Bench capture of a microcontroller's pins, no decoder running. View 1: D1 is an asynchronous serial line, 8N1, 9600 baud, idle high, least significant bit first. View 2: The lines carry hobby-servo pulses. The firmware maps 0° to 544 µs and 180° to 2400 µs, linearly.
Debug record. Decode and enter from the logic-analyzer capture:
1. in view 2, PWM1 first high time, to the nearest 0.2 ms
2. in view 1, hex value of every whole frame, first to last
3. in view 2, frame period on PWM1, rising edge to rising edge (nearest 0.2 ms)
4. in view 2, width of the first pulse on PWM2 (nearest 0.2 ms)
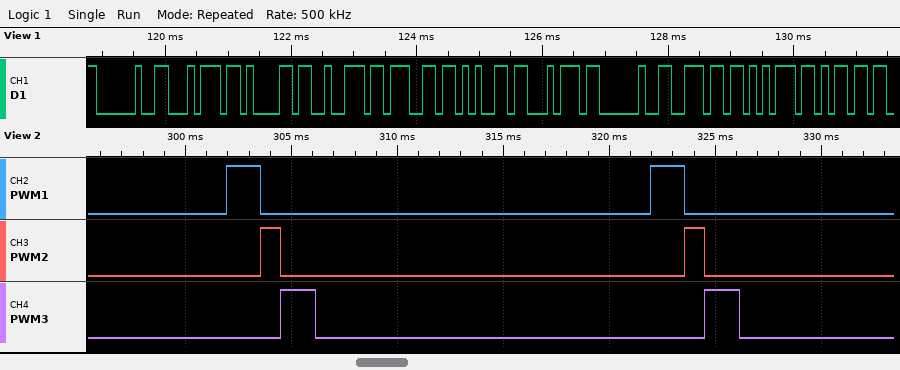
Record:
1.6 ms
0x20 0x74 0x61 0x72 0x67 0x65 0x74 0x20 0x6E 0x75 0x6D
20.0 ms
1.0 ms
